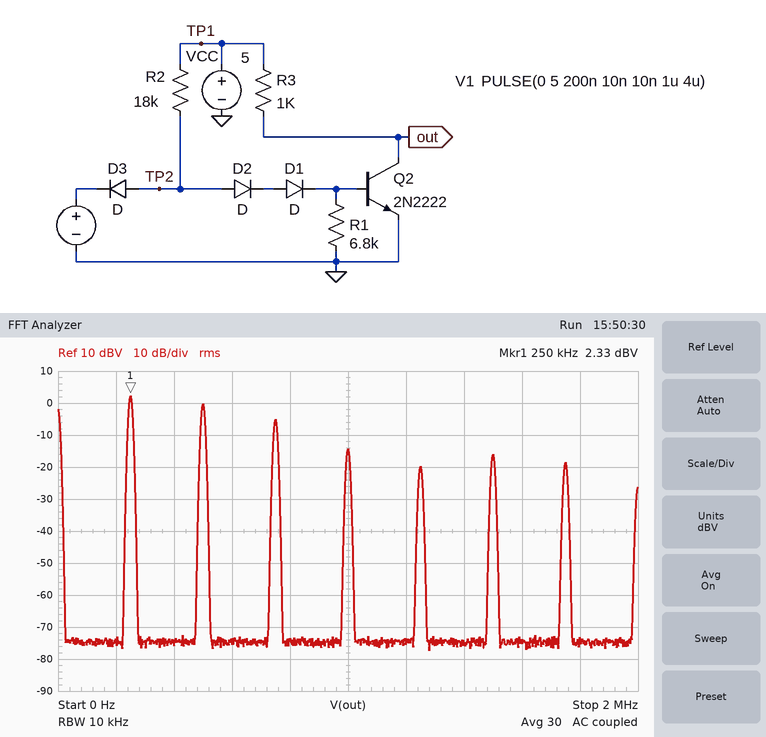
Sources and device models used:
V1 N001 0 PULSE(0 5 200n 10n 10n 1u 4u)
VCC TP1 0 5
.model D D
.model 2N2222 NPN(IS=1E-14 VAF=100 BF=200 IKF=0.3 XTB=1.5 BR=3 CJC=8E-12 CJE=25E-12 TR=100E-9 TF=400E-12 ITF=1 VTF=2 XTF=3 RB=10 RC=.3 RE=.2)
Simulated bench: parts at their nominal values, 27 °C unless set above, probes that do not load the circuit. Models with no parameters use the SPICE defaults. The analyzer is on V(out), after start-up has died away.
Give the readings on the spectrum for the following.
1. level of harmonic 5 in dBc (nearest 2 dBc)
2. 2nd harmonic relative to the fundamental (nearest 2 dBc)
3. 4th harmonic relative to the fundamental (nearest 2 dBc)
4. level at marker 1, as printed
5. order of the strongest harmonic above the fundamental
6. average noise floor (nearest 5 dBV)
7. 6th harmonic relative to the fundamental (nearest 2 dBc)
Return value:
-22 dBc
-2 dBc
-16 dBc
2.33 dBV
2
-75 dBV
-18 dBc
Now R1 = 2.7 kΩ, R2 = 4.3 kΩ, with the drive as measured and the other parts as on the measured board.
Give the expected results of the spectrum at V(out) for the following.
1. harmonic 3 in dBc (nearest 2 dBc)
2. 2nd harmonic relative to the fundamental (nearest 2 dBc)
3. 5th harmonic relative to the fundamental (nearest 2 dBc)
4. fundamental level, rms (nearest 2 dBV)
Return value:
-26 dBc
-6 dBc
-14 dBc
6 dBV
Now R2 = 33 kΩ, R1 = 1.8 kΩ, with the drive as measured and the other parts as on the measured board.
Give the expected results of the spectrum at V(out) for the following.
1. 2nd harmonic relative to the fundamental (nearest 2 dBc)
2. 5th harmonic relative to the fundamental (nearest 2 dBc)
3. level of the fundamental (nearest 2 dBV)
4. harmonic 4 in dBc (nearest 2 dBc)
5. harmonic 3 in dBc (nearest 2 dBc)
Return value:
2 dBc
0 dBc
-68 dBV
-22 dBc
0 dBc
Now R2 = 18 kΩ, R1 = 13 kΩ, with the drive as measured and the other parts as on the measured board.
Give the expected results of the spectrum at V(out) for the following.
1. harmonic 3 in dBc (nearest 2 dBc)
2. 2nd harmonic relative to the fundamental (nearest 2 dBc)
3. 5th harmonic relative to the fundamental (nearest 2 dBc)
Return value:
-20 dBc
-6 dBc
-16 dBc
